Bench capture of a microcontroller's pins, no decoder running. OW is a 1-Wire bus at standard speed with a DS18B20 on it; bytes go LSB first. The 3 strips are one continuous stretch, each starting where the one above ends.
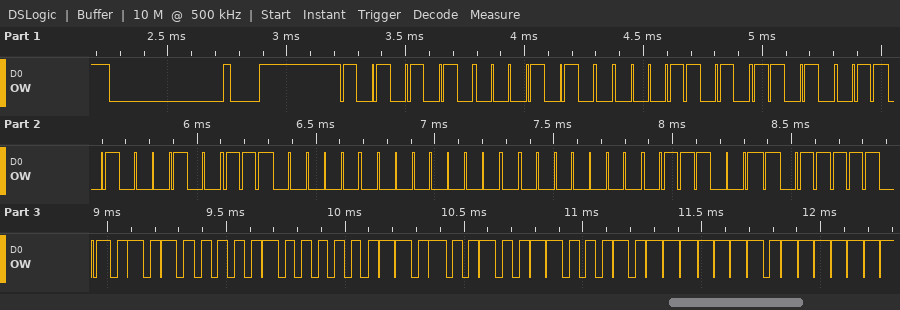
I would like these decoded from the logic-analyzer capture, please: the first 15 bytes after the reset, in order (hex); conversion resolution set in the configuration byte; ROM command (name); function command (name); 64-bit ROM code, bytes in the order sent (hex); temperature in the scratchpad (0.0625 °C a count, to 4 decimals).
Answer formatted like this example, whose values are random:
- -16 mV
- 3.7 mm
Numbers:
- 55 28 58 CB 22 07 00 00 CE BE 0A 02 4B 46 7F
- 12 bits
- Match ROM
- Read Scratchpad
- 28 58 CB 22 07 00 00 CE
- 32.6250 °C
